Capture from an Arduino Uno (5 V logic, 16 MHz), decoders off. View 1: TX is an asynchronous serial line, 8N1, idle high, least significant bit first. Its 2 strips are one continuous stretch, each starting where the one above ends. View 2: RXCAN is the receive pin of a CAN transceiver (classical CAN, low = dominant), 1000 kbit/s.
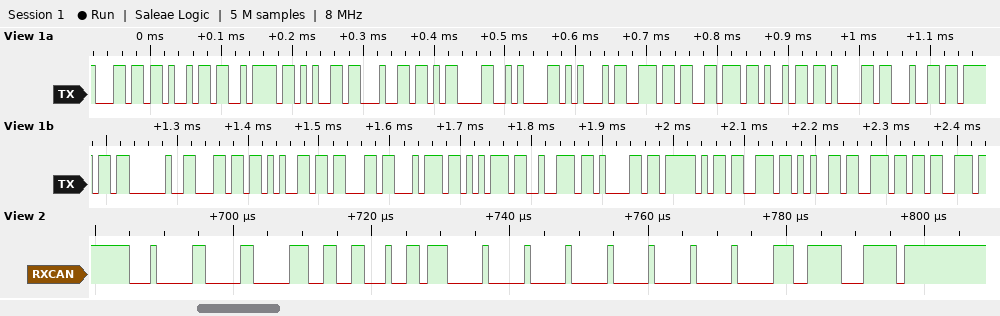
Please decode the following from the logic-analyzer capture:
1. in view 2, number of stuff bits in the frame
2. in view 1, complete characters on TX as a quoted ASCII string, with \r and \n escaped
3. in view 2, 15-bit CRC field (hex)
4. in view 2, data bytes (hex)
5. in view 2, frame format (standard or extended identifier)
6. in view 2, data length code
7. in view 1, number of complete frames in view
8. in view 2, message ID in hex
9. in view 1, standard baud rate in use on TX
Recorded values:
12
"lized\r\nEnviado lectura_sens"
0x67CF
33 31 37 00 00 00 00 00
standard
8
27
0x104
115200 baud
